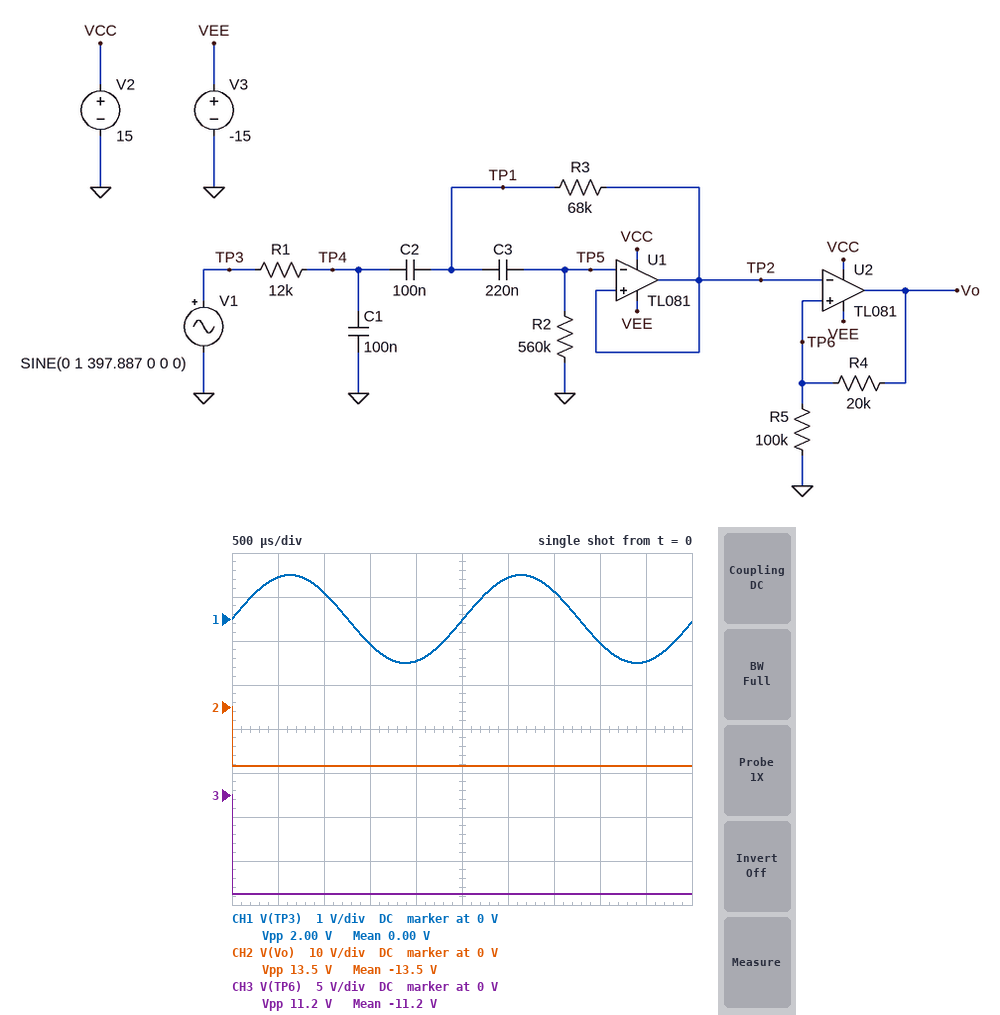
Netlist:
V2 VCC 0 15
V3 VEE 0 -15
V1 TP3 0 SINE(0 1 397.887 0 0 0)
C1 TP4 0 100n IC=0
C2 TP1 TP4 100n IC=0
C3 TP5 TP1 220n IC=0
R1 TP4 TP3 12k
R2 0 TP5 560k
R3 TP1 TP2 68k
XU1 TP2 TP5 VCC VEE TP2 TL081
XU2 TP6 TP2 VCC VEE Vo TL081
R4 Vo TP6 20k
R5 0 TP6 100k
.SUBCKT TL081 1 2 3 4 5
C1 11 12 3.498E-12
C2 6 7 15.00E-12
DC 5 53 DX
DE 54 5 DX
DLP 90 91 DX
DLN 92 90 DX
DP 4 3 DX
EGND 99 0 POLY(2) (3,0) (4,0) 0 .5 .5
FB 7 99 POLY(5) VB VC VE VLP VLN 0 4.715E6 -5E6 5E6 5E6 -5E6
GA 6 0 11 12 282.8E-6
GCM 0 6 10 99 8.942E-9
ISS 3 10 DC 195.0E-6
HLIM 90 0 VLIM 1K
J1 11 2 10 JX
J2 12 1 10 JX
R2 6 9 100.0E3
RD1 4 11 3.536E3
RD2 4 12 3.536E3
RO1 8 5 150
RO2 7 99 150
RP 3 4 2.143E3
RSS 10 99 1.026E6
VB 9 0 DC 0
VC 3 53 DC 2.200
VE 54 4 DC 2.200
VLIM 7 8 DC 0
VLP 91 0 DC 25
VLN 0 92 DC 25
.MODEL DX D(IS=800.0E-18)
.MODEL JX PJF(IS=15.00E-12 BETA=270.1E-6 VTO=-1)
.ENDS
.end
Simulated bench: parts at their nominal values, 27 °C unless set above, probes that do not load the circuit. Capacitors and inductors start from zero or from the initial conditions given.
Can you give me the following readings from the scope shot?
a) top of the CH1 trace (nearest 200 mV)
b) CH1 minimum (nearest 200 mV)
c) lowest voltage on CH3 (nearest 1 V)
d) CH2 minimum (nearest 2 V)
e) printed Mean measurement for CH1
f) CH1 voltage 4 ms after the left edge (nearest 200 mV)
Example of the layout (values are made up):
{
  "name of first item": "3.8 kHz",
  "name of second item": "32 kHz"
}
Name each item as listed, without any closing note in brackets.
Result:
{
  "top of the CH1 trace": "1.0 V",
  "CH1 minimum": "-1.0 V",
  "lowest voltage on CH3": "-11 V",
  "CH2 minimum": "-14 V",
  "printed Mean measurement for CH1": "0.00 V",
  "CH1 voltage 4 ms after the left edge": "-600 mV"
}
